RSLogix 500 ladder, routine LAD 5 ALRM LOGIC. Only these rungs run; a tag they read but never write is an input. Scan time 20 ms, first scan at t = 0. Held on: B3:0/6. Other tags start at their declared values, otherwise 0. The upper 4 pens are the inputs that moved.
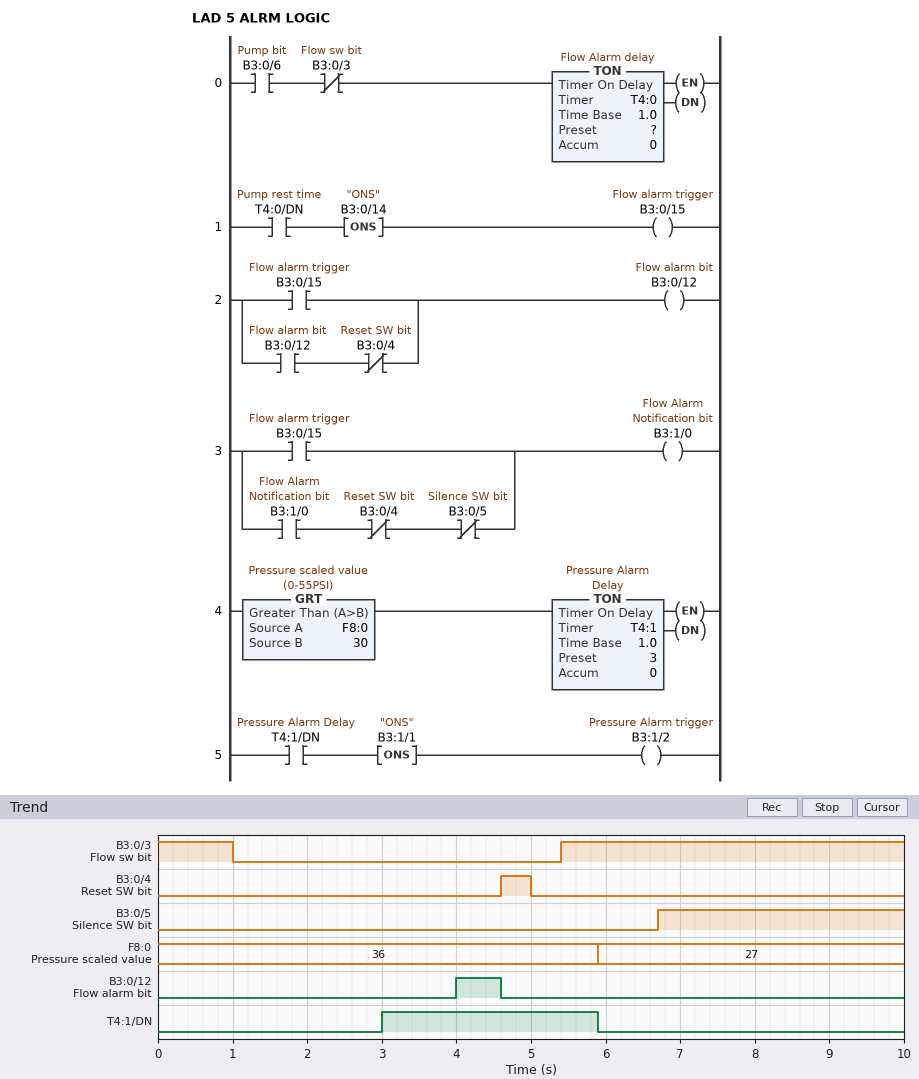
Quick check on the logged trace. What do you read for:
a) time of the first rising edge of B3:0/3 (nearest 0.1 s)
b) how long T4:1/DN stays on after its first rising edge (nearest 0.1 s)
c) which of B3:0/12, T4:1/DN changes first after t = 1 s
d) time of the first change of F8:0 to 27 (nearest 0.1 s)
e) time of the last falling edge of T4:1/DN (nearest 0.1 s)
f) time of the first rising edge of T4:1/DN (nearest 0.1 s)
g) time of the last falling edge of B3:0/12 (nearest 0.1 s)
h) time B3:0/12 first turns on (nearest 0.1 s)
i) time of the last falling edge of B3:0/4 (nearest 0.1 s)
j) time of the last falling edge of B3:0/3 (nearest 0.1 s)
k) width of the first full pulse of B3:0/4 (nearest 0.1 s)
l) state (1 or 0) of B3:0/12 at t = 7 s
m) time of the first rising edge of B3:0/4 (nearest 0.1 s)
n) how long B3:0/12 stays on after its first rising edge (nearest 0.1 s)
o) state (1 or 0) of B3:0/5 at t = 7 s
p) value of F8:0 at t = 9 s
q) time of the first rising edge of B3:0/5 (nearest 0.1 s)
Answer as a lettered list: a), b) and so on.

a) 5.4 s
b) 2.9 s
c) T4:1/DN
d) 5.9 s
e) 5.9 s
f) 3.0 s
g) 4.6 s
h) 4.0 s
i) 5.0 s
j) 1.0 s
k) 0.4 s
l) 0
m) 4.6 s
n) 0.6 s
o) 1
p) 27
q) 6.7 s
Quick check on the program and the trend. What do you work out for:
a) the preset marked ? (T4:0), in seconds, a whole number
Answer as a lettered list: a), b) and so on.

a) 3 s
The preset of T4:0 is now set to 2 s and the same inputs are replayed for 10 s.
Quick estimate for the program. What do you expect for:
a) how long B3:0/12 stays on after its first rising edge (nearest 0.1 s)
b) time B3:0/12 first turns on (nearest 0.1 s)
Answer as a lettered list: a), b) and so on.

a) 1.6 s
b) 3.0 s
